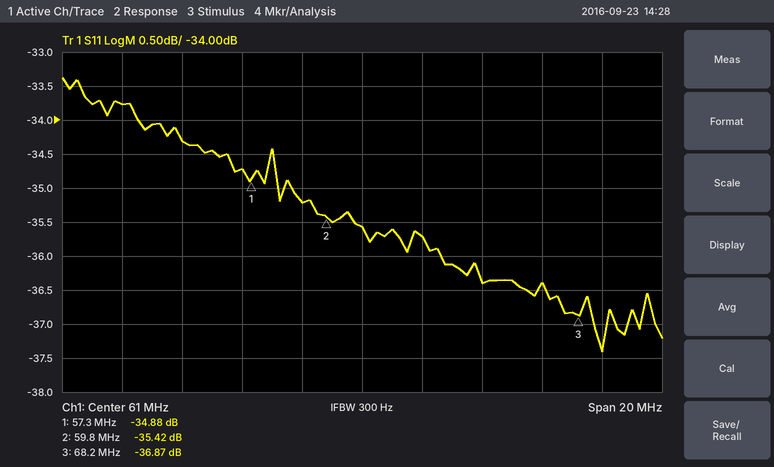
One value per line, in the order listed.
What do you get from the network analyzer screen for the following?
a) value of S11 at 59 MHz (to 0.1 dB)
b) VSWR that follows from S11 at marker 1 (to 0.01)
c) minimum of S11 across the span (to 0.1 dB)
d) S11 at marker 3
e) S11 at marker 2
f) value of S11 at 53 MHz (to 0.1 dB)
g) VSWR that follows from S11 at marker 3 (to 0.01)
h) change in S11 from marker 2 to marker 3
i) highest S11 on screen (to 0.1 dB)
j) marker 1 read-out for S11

-35.2 dB
1.04
-37.4 dB
-36.87 dB
-35.42 dB
-33.8 dB
1.03
-1.45 dB
-33.4 dB
-34.88 dB
